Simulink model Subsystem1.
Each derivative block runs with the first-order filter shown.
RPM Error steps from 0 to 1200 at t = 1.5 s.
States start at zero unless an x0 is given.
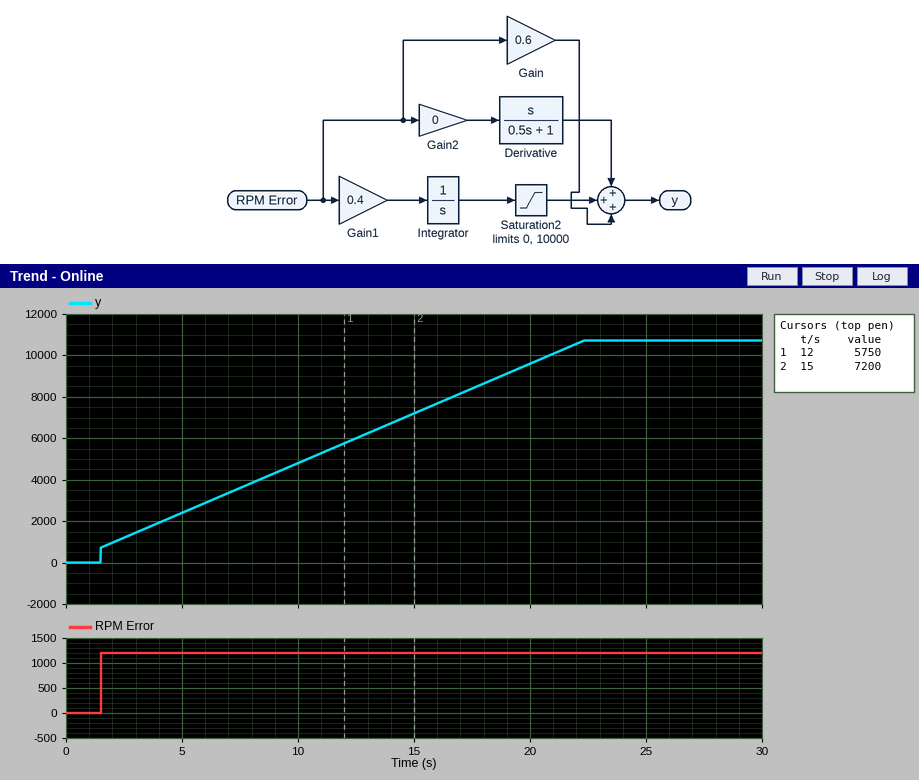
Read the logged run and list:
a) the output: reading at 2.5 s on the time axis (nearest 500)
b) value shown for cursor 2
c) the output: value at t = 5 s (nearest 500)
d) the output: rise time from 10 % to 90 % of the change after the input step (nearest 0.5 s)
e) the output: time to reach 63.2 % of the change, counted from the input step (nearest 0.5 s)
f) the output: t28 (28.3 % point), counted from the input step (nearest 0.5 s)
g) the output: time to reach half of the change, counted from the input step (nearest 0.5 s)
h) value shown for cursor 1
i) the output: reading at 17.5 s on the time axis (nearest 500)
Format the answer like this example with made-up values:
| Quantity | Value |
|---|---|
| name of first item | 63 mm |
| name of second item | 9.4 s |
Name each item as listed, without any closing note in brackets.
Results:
| Quantity | Value |
|---|---|
| the output: reading at 2.5 s on the time axis | 1000 |
| value shown for cursor 2 | 7200 |
| the output: value at t = 5 s | 2500 |
| the output: rise time from 10 % to 90 % of the change after the input step | 18.0 s |
| the output: time to reach 63.2 % of the change, counted from the input step | 12.5 s |
| the output: t28 (28.3 % point), counted from the input step | 5.0 s |
| the output: time to reach half of the change, counted from the input step | 9.5 s |
| value shown for cursor 1 | 5750 |
| the output: reading at 17.5 s on the time axis | 8500 |
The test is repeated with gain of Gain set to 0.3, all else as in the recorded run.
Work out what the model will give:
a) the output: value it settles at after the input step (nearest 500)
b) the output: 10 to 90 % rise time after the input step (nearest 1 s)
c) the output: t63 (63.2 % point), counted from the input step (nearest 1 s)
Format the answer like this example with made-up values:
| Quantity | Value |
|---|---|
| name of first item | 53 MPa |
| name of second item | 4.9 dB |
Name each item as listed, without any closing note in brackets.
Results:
| Quantity | Value |
|---|---|
| the output: value it settles at after the input step | 10500 |
| the output: 10 to 90 % rise time after the input step | 17 s |
| the output: t63 (63.2 % point), counted from the input step | 13 s |
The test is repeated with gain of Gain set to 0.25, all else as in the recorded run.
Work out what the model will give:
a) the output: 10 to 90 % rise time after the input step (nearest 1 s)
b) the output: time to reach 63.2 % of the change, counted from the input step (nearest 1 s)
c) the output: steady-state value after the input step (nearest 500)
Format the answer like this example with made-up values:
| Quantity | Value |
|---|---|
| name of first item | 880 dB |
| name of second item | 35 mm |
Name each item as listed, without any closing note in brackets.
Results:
| Quantity | Value |
|---|---|
| the output: 10 to 90 % rise time after the input step | 17 s |
| the output: time to reach 63.2 % of the change, counted from the input step | 13 s |
| the output: steady-state value after the input step | 10500 |
